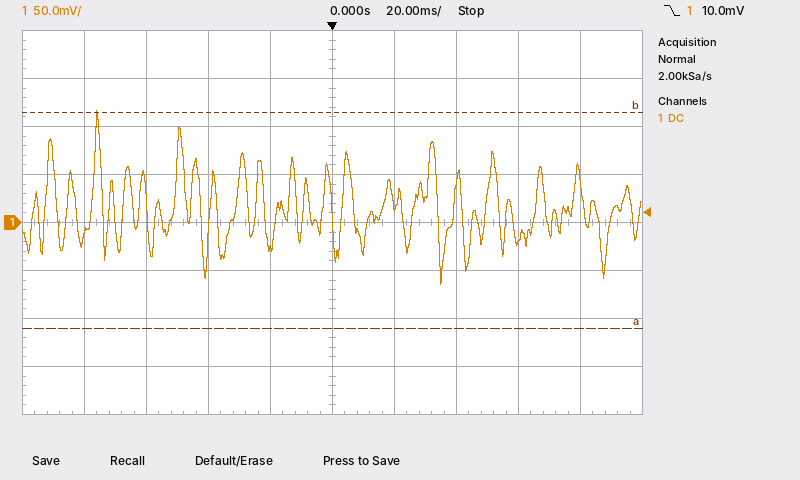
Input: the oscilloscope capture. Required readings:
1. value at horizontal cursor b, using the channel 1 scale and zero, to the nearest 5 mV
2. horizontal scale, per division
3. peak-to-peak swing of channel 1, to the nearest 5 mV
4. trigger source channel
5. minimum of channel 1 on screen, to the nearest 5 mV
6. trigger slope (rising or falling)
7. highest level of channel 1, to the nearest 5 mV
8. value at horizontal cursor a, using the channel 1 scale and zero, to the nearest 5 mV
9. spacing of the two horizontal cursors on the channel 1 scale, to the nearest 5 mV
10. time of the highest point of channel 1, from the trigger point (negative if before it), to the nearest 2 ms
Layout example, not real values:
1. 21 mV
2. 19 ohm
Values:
1. 115 mV
2. 20 ms
3. 180 mV
4. channel 1
5. -65 mV
6. falling
7. 115 mV
8. -110 mV
9. 225 mV
10. -76 ms
